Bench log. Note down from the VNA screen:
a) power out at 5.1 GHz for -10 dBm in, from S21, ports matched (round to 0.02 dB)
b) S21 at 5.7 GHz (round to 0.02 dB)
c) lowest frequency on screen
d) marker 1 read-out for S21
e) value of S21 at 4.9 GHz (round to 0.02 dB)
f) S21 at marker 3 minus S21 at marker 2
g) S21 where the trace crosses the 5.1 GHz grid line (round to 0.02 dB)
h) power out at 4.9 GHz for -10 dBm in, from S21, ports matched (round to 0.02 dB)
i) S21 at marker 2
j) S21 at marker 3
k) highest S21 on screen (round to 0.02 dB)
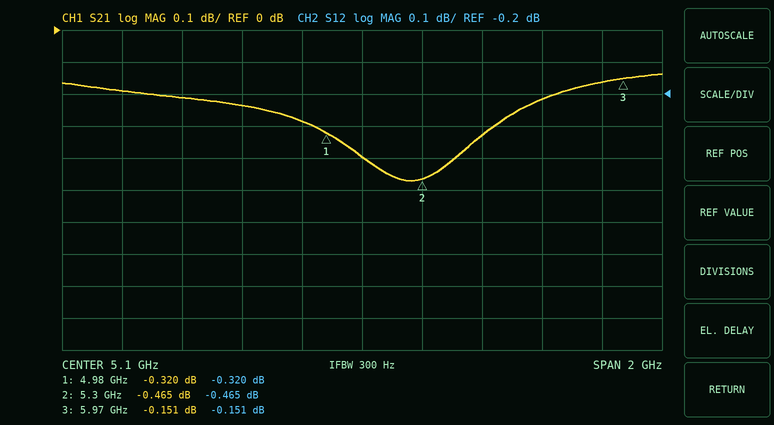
-10.40 dBm
-0.22 dB
4.1 GHz
-0.320 dB
-0.28 dB
0.314 dB
-0.40 dB
-10.28 dBm
-0.465 dB
-0.151 dB
-0.14 dB
